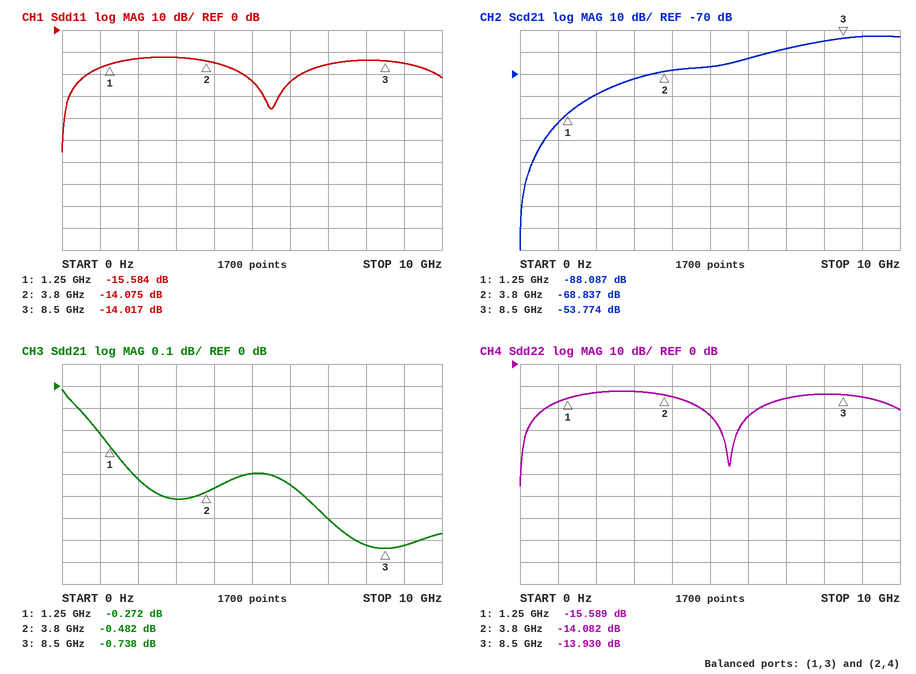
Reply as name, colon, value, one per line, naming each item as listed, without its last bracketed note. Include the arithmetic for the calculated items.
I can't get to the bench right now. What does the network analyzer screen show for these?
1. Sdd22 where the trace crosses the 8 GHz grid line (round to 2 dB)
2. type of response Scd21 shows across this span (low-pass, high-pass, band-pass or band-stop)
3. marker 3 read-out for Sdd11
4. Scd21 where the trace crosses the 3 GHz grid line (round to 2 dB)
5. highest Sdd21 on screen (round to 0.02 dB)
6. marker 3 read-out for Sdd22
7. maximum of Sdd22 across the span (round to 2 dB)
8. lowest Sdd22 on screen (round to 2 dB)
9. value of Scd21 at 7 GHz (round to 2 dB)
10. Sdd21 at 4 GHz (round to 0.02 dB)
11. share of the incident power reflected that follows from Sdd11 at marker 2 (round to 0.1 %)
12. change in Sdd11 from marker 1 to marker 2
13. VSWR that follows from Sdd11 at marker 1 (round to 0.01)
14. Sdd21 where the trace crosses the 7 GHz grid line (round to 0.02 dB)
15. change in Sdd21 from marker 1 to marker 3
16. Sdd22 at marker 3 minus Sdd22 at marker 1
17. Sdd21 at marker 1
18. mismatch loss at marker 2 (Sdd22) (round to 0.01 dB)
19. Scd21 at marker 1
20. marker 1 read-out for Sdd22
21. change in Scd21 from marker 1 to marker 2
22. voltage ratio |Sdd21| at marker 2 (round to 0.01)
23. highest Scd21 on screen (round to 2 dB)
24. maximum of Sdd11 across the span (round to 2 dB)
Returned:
Sdd22 where the trace crosses the 8 GHz grid line: -14 dB
type of response Scd21 shows across this span: high-pass
marker 3 read-out for Sdd11: -14.017 dB
Scd21 where the trace crosses the 3 GHz grid line: -72 dB
highest Sdd21 on screen: -0.02 dB
marker 3 read-out for Sdd22: -13.930 dB
maximum of Sdd22 across the span: -12 dB
lowest Sdd22 on screen: -56 dB
value of Scd21 at 7 GHz: -58 dB
Sdd21 at 4 GHz: -0.46 dB
share of the incident power reflected that follows from Sdd11 at marker 2: 10^(-14.075/10) ≈ 3.9 %
change in Sdd11 from marker 1 to marker 2: -14.075 − (-15.584) = 1.509 dB
VSWR that follows from Sdd11 at marker 1: (1 + 0.1663)/(1 − 0.1663) ≈ 1.40
Sdd21 where the trace crosses the 7 GHz grid line: -0.60 dB
change in Sdd21 from marker 1 to marker 3: -0.738 − (-0.272) = -0.466 dB
Sdd22 at marker 3 minus Sdd22 at marker 1: -13.93 − (-15.589) = 1.659 dB
Sdd21 at marker 1: -0.272 dB
mismatch loss at marker 2 (Sdd22): −10 log10(1 − 10^(-14.082/10)) ≈ 0.17 dB
Scd21 at marker 1: -88.087 dB
marker 1 read-out for Sdd22: -15.589 dB
change in Scd21 from marker 1 to marker 2: -68.837 − (-88.087) = 19.250 dB
voltage ratio |Sdd21| at marker 2: 10^(-0.482/20) ≈ 0.95
highest Scd21 on screen: -52 dB
maximum of Sdd11 across the span: -12 dB
